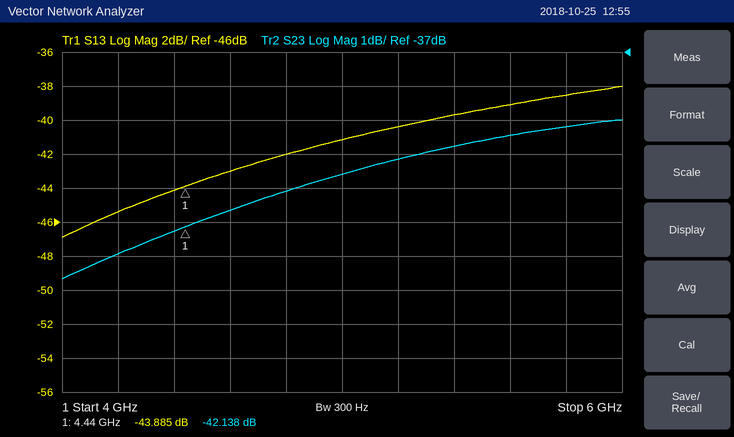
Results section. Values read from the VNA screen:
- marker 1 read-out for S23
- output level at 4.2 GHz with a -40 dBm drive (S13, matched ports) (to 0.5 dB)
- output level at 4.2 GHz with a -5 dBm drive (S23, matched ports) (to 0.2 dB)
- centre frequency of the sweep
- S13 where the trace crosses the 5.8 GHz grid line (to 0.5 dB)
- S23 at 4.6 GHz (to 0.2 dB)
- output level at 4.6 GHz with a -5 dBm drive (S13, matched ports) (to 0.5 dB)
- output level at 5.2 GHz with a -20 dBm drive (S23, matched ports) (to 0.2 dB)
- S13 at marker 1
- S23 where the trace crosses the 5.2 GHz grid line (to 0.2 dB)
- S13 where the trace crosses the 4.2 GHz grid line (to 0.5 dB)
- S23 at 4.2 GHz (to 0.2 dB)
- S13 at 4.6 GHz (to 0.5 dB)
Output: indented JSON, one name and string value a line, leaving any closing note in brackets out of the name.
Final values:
{
  "marker 1 read-out for S23": "-42.138 dB",
  "output level at 4.2 GHz with a -40 dBm drive (S13, matched ports)": "-85.5 dBm",
  "output level at 4.2 GHz with a -5 dBm drive (S23, matched ports)": "-48.0 dBm",
  "centre frequency of the sweep": "5 GHz",
  "S13 where the trace crosses the 5.8 GHz grid line": "-38.5 dB",
  "S23 at 4.6 GHz": "-41.6 dB",
  "output level at 4.6 GHz with a -5 dBm drive (S13, matched ports)": "-48.0 dBm",
  "output level at 5.2 GHz with a -20 dBm drive (S23, matched ports)": "-60.2 dBm",
  "S13 at marker 1": "-43.885 dB",
  "S23 where the trace crosses the 5.2 GHz grid line": "-40.2 dB",
  "S13 where the trace crosses the 4.2 GHz grid line": "-45.5 dB",
  "S23 at 4.2 GHz": "-43.0 dB",
  "S13 at 4.6 GHz": "-43.0 dB"
}
